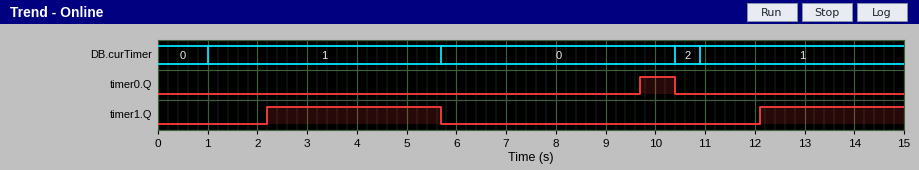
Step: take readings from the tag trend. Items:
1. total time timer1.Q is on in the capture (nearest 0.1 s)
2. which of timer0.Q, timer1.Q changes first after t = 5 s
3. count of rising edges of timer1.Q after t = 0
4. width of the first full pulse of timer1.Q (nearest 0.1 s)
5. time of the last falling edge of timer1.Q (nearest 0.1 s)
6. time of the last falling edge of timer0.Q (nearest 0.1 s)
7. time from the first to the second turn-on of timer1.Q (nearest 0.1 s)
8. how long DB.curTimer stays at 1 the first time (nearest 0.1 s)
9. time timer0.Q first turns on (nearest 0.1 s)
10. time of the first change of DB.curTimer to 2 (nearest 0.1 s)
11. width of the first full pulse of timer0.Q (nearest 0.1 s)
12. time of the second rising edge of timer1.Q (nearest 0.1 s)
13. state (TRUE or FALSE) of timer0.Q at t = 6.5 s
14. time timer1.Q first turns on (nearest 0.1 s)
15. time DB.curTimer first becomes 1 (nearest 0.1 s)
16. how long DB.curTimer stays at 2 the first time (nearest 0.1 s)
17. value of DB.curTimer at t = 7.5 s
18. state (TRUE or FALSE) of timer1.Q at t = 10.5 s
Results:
6.4 s
timer1.Q
2
3.5 s
5.7 s
10.4 s
9.9 s
4.7 s
9.7 s
10.4 s
0.7 s
12.1 s
FALSE
2.2 s
1.0 s
0.5 s
0
FALSE
